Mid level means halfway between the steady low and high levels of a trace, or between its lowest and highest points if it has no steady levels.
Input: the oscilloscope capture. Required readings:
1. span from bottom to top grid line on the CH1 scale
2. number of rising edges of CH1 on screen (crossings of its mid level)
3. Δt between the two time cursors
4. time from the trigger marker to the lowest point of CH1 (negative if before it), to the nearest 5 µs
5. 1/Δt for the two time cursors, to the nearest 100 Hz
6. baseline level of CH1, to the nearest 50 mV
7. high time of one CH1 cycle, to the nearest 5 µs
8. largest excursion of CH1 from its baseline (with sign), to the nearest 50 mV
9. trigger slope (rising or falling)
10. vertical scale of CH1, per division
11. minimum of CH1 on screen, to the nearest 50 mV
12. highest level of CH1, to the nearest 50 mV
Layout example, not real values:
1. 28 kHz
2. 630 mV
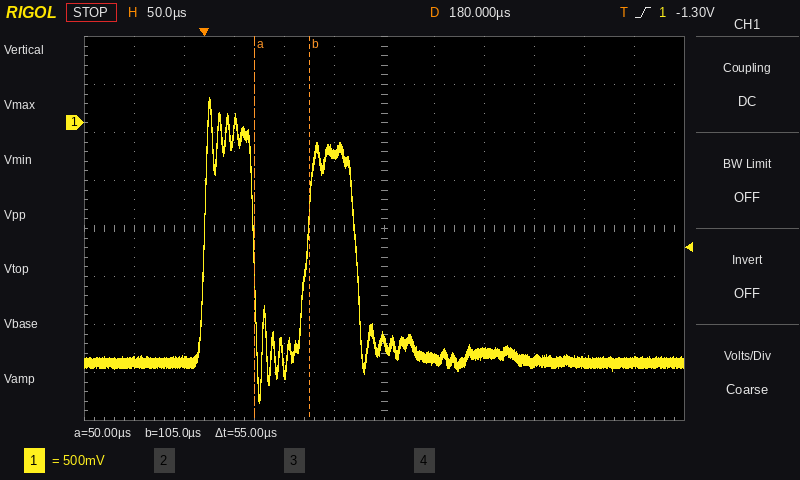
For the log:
1. 4 V
2. 2
3. 55 µs
4. +55 µs
5. 18.2 kHz
6. -2.50 V
7. 50 µs
8. +2.75 V
9. rising
10. 500 mV
11. -2.90 V
12. 250 mV
